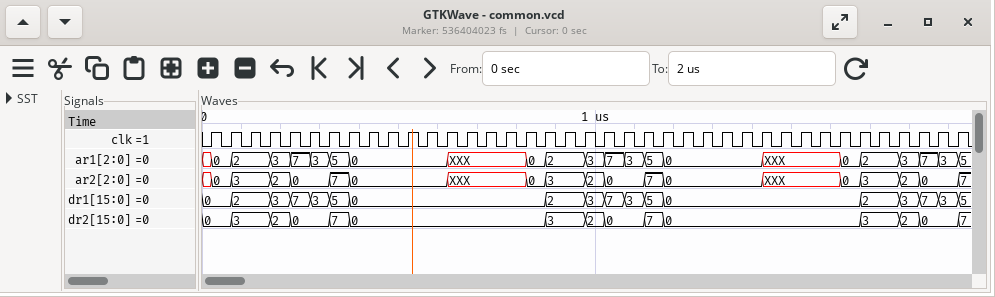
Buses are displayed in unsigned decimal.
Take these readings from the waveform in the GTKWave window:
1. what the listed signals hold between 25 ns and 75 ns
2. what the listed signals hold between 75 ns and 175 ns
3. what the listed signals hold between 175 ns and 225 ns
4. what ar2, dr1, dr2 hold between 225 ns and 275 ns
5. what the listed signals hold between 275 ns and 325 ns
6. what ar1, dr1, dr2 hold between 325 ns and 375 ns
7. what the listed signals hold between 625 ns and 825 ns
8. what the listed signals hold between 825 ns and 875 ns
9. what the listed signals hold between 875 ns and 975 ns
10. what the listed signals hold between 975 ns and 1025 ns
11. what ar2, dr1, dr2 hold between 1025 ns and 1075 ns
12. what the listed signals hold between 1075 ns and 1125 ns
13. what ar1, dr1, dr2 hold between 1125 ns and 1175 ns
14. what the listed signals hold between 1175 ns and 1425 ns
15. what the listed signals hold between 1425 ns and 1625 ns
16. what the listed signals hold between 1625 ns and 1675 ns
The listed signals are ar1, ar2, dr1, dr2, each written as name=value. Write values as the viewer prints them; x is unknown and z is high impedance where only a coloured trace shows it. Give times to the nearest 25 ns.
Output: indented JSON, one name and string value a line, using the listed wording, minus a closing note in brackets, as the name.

{
  "what the listed signals hold between 25 ns and 75 ns": "ar1=0, ar2=0, dr1=0, dr2=0",
  "what the listed signals hold between 75 ns and 175 ns": "ar1=2, ar2=3, dr1=2, dr2=3",
  "what the listed signals hold between 175 ns and 225 ns": "ar1=3, ar2=2, dr1=3, dr2=2",
  "what ar2, dr1, dr2 hold between 225 ns and 275 ns": "ar2=0, dr1=7, dr2=0",
  "what the listed signals hold between 275 ns and 325 ns": "ar1=3, ar2=0, dr1=3, dr2=0",
  "what ar1, dr1, dr2 hold between 325 ns and 375 ns": "ar1=5, dr1=5, dr2=7",
  "what the listed signals hold between 625 ns and 825 ns": "ar1=XXX, ar2=XXX, dr1=0, dr2=0",
  "what the listed signals hold between 825 ns and 875 ns": "ar1=0, ar2=0, dr1=0, dr2=0",
  "what the listed signals hold between 875 ns and 975 ns": "ar1=2, ar2=3, dr1=2, dr2=3",
  "what the listed signals hold between 975 ns and 1025 ns": "ar1=3, ar2=2, dr1=3, dr2=2",
  "what ar2, dr1, dr2 hold between 1025 ns and 1075 ns": "ar2=0, dr1=7, dr2=0",
  "what the listed signals hold between 1075 ns and 1125 ns": "ar1=3, ar2=0, dr1=3, dr2=0",
  "what ar1, dr1, dr2 hold between 1125 ns and 1175 ns": "ar1=5, dr1=5, dr2=7",
  "what the listed signals hold between 1175 ns and 1425 ns": "ar1=0, ar2=0, dr1=0, dr2=0",
  "what the listed signals hold between 1425 ns and 1625 ns": "ar1=XXX, ar2=XXX, dr1=0, dr2=0",
  "what the listed signals hold between 1625 ns and 1675 ns": "ar1=0, ar2=0, dr1=0, dr2=0"
}
